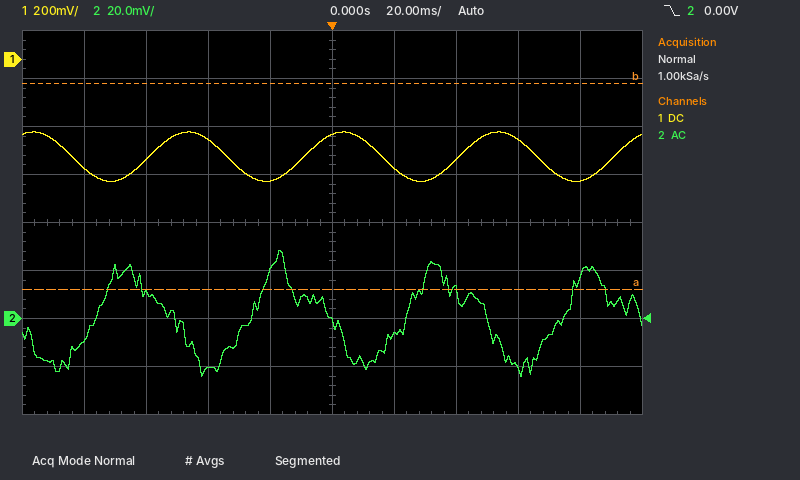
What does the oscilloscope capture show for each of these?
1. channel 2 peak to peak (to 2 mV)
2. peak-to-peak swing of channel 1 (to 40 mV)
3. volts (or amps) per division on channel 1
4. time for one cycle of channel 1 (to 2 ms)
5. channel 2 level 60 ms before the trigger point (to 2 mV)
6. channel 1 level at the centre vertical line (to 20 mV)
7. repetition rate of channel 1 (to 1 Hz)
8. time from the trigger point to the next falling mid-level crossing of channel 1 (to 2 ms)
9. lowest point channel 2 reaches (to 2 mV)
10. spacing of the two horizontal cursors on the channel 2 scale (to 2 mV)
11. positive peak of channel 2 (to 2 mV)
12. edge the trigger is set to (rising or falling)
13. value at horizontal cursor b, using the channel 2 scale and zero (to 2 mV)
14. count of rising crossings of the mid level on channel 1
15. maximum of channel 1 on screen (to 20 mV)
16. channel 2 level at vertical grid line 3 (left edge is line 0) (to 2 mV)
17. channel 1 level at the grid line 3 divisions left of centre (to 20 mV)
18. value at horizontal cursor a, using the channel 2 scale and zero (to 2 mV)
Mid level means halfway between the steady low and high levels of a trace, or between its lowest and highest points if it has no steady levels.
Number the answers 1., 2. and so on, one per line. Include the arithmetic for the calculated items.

1. 28 mV − (-24 mV) = 52 mV
2. 200 mV
3. 200 mV
4. 50 ms
5. 10 mV
6. -320 mV
7. 1 / 50 ms ≈ 20 Hz
8. 16 ms
9. -24 mV
10. 86 mV
11. 28 mV
12. falling
13. 98 mV
14. 4
15. -300 mV
16. -20 mV
17. -420 mV
18. 12 mV
